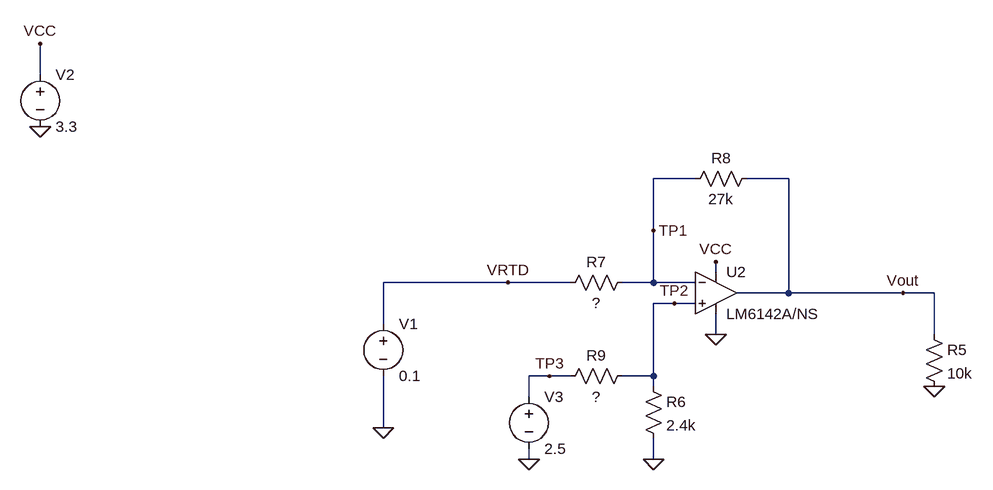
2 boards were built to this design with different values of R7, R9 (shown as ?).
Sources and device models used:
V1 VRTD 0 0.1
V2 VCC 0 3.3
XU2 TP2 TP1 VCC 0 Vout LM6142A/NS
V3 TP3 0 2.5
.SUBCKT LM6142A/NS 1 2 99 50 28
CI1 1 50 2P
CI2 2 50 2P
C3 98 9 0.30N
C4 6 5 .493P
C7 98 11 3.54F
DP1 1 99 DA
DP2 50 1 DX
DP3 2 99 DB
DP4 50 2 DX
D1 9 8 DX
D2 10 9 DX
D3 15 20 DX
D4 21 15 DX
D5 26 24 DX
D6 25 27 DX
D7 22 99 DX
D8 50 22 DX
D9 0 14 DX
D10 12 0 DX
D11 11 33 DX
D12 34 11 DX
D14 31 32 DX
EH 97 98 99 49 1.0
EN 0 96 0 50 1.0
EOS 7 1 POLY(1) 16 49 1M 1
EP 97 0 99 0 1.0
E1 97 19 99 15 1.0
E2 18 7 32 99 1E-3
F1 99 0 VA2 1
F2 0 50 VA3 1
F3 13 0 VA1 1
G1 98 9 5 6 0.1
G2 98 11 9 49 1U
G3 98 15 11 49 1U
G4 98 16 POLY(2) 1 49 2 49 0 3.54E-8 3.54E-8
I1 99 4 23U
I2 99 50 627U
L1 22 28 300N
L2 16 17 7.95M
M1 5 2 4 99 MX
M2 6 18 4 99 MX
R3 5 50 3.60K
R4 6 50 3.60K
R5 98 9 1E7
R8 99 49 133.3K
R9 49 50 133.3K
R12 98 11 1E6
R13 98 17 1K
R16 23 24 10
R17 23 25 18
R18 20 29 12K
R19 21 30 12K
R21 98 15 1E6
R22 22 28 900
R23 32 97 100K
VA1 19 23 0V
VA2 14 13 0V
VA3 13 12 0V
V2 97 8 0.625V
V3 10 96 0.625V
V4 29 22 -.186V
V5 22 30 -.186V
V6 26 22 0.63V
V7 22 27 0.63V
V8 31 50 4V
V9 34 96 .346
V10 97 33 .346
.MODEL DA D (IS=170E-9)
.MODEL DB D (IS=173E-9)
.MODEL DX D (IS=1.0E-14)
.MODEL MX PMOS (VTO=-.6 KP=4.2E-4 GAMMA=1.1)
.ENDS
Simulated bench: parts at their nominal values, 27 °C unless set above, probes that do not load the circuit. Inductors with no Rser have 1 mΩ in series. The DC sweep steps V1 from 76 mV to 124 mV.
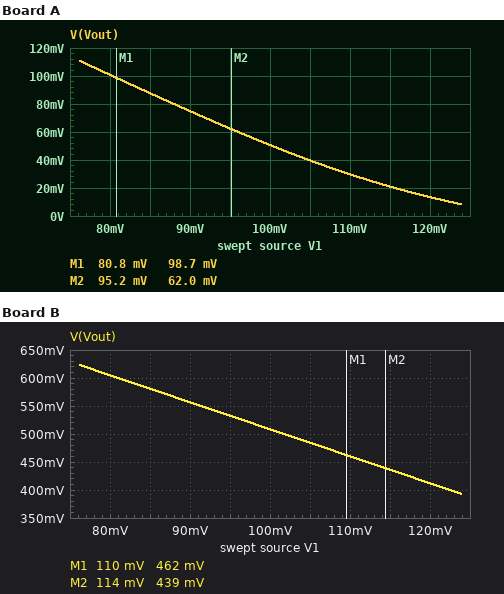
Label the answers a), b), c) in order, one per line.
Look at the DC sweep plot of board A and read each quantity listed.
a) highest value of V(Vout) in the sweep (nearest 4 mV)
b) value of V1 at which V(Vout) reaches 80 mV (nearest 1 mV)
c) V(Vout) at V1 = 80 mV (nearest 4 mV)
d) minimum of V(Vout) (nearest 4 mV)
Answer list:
a) 112 mV
b) 88 mV
c) 100 mV
d) 8 mV
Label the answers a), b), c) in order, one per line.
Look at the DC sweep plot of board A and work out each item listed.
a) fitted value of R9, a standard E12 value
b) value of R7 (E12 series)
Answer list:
a) 68 kΩ
b) 10 kΩ
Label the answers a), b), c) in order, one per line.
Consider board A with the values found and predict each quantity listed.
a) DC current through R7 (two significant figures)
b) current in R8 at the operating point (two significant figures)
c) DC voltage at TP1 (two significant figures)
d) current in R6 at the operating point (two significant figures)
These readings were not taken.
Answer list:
a) 1.2 µA
b) 1.4 µA
c) 88 mV
d) 36 µA
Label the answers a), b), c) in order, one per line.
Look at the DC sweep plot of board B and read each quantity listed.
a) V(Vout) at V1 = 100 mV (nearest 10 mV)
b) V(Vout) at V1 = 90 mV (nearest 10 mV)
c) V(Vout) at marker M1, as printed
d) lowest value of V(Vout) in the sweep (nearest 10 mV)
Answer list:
a) 510 mV
b) 560 mV
c) 462 mV
d) 390 mV
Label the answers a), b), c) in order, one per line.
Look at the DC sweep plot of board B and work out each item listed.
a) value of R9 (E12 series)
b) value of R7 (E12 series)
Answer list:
a) 33 kΩ
b) 5.6 kΩ
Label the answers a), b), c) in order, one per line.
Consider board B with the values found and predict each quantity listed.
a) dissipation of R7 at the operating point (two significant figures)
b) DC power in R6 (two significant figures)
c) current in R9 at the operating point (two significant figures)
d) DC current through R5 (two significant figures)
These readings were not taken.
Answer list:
a) 900 nW
b) 12 µW
c) 71 µA
d) 51 µA
